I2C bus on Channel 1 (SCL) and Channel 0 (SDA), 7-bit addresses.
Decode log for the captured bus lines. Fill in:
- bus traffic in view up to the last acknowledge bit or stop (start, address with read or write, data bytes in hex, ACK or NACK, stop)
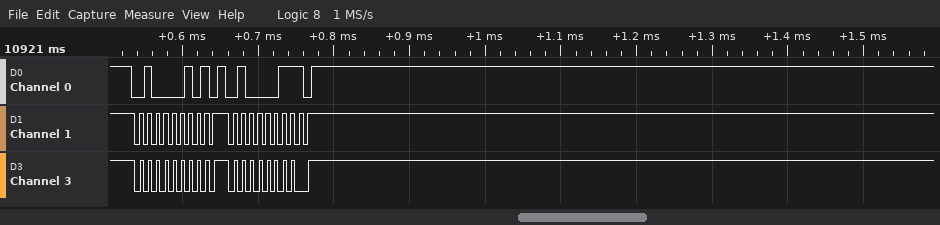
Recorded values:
start, address 21 write NACK, stop, start, address 21 read NACK, stop
